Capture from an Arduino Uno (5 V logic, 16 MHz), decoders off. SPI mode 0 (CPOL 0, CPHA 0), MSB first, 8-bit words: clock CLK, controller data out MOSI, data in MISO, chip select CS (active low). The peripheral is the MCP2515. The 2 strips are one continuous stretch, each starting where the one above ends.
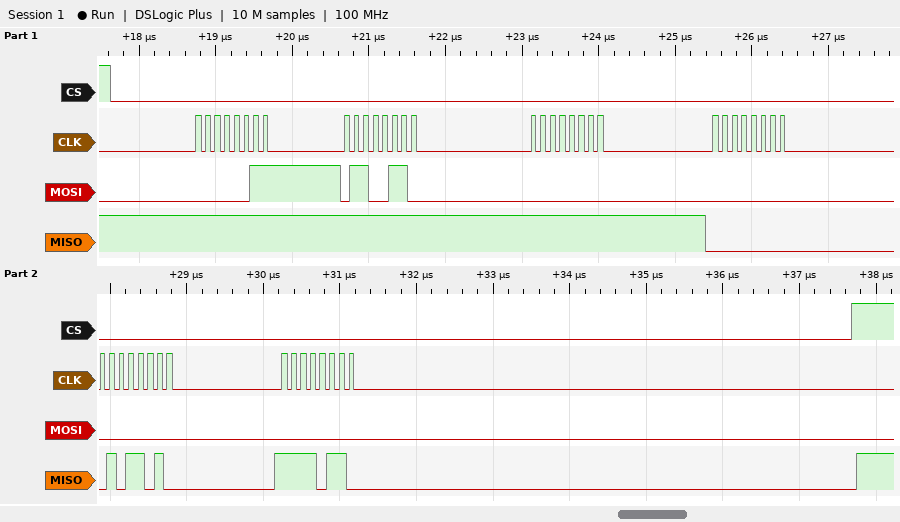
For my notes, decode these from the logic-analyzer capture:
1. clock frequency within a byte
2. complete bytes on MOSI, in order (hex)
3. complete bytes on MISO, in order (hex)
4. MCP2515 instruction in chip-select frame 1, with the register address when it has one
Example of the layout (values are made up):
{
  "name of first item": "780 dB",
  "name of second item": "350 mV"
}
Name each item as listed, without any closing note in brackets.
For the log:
{
  "clock frequency within a byte": "8 MHz",
  "complete bytes on MOSI, in order": "03 66 00 00 00 00",
  "complete bytes on MISO, in order": "FF FF FF 00 5A F6",
  "MCP2515 instruction in chip-select frame 1, with the register address when it has one": "READ 0x66"
}
